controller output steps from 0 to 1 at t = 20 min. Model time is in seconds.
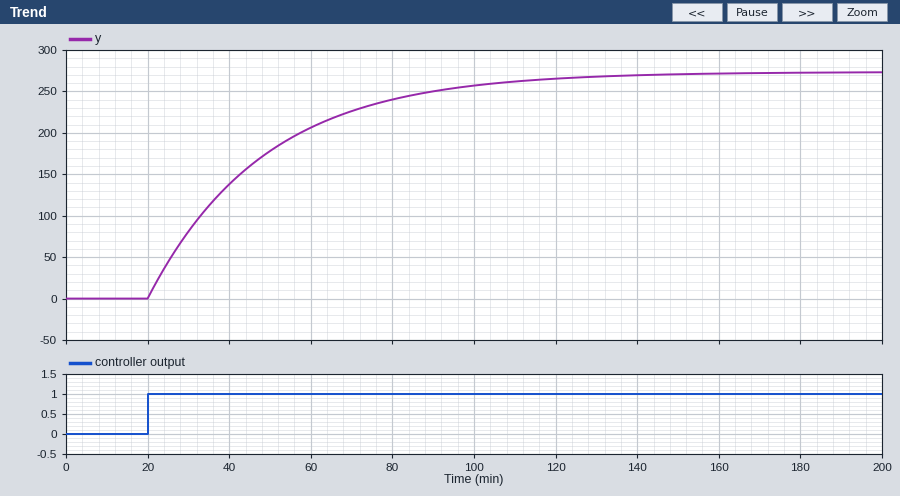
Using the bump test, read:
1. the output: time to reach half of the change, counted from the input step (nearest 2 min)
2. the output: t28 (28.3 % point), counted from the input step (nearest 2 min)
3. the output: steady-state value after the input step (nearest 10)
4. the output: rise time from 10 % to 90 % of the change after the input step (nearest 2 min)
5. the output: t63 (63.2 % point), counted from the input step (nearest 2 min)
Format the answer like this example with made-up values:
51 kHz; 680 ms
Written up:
20 min; 10 min; 270; 62 min; 28 min
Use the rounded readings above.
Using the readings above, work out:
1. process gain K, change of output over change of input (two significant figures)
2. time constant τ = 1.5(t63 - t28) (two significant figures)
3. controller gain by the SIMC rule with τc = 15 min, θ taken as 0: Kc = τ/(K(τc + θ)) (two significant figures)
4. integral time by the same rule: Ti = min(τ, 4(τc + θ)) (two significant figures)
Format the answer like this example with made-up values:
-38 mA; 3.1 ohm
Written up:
270; 27 min; 0.0067; 27 min
